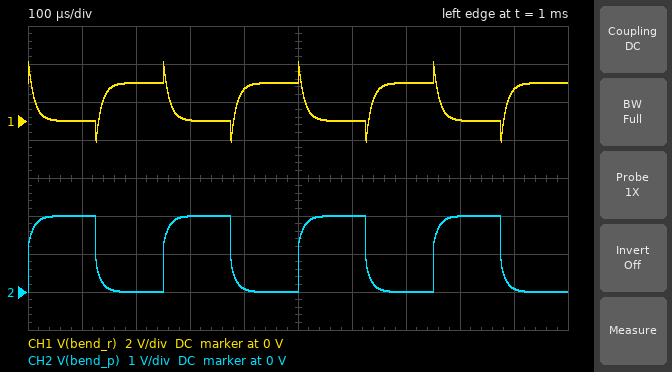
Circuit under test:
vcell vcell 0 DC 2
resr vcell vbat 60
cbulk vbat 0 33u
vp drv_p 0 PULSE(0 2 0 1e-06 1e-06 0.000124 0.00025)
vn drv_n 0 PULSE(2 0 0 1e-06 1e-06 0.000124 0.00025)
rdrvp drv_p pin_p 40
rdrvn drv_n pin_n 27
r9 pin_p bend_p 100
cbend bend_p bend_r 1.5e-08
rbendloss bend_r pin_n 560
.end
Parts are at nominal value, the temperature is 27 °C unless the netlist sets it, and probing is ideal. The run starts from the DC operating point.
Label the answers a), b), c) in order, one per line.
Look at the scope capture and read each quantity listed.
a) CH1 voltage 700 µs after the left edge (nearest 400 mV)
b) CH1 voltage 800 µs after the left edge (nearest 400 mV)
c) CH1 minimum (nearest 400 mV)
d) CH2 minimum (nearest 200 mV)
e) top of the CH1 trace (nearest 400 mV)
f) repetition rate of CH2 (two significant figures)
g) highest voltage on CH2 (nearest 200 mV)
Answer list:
a) 2.0 V
b) 0 V
c) -1.2 V
d) 0 V
e) 3.2 V
f) 4.0 kHz
g) 2.0 V
